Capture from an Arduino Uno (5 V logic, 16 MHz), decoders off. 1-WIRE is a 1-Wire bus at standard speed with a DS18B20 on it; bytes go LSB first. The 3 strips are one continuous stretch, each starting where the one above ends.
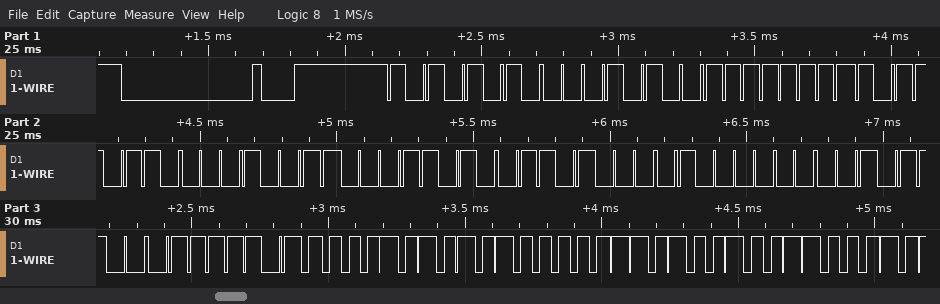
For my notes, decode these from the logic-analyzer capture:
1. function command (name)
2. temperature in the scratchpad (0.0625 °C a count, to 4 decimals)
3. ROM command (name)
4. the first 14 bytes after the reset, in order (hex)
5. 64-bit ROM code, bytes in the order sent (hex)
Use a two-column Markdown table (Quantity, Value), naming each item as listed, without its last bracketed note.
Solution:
| Quantity | Value |
|---|---|
| function command | Read Scratchpad |
| temperature in the scratchpad | 85.0000 °C |
| ROM command | Match ROM |
| the first 14 bytes after the reset, in order | 55 28 FF 6D C8 58 16 02 34 BE 50 05 4B 46 |
| 64-bit ROM code, bytes in the order sent | 28 FF 6D C8 58 16 02 34 |
